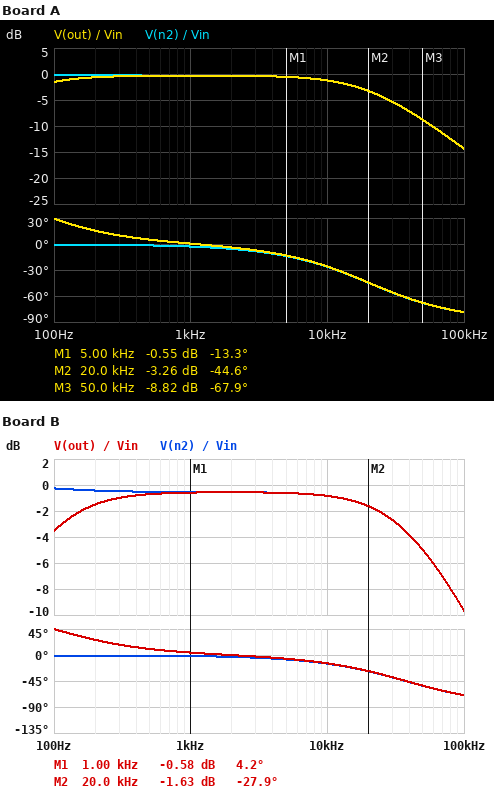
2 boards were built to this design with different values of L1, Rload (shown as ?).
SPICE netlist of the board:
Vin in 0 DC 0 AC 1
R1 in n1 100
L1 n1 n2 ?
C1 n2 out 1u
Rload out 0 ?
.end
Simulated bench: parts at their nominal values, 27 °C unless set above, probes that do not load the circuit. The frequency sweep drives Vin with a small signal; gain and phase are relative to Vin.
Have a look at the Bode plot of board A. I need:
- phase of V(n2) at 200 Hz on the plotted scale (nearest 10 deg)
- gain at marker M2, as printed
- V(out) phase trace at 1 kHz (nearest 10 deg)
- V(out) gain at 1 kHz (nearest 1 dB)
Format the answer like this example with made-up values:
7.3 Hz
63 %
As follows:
0 deg
-3.26 dB
0 deg
0 dB
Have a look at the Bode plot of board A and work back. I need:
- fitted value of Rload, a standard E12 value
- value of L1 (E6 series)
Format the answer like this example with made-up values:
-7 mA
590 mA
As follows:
2.7 kΩ
22 mH
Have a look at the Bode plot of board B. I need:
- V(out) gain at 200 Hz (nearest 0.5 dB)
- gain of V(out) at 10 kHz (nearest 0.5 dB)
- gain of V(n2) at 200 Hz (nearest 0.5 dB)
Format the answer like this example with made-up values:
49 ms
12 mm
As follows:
-1.5 dB
-1.0 dB
-0.5 dB
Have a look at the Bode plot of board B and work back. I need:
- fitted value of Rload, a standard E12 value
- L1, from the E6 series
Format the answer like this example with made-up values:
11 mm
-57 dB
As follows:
1.5 kΩ
6.8 mH
